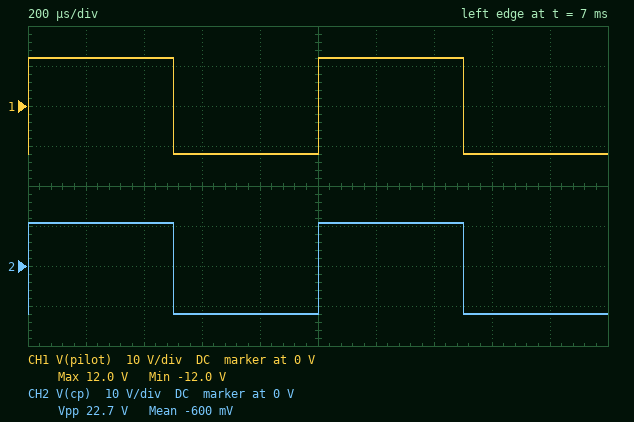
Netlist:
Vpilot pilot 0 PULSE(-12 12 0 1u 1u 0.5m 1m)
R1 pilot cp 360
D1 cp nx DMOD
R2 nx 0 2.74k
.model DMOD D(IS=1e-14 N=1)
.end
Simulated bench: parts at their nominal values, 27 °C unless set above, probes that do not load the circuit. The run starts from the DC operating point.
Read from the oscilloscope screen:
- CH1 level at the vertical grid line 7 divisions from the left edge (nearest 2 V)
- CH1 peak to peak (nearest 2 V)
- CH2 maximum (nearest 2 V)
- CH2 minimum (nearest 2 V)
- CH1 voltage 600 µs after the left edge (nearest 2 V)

12 V
24 V
10 V
-12 V
-12 V
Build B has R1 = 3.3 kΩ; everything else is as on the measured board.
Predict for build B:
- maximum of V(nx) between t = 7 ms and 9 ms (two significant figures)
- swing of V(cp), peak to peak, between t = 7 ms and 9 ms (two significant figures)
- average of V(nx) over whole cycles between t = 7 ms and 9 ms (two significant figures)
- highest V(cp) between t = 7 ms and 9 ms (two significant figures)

5.1 V
18 V
2.6 V
5.8 V
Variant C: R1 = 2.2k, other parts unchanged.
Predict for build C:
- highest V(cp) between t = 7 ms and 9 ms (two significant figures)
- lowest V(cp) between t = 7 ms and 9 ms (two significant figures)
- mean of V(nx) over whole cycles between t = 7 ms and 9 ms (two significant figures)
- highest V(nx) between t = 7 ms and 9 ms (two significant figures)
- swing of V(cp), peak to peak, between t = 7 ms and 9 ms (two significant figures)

7.0 V
-12 V
3.1 V
6.3 V
19 V
